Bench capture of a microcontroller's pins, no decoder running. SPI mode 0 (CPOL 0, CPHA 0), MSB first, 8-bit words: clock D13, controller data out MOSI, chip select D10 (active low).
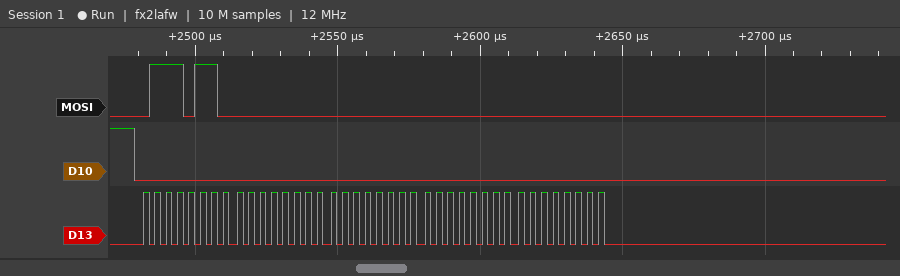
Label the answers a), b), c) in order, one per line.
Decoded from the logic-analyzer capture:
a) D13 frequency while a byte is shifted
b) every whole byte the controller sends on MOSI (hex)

a) 250 kHz
b) 76 00 00 00 00
